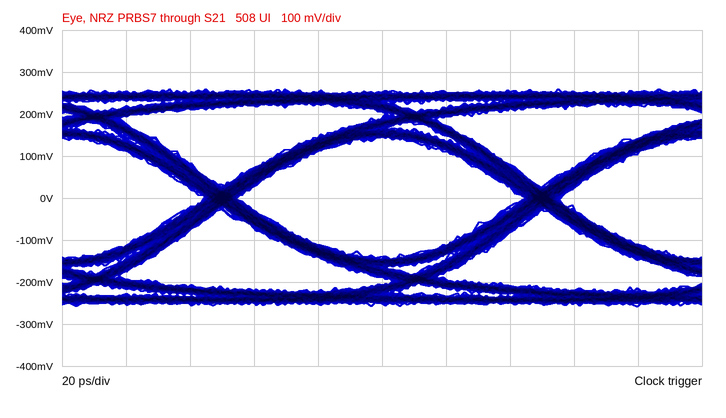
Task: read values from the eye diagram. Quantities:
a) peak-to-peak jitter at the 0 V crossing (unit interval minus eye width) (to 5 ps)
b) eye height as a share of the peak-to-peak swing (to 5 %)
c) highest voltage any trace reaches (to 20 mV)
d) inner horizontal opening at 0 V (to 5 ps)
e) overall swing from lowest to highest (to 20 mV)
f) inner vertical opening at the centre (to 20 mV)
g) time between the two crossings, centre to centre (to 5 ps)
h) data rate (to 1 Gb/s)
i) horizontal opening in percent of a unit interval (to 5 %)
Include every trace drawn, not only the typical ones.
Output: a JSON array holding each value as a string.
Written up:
["10 ps", "55 %", "260 mV", "90 ps", "520 mV", "280 mV", "100 ps", "10 Gb/s", "90 %"]
